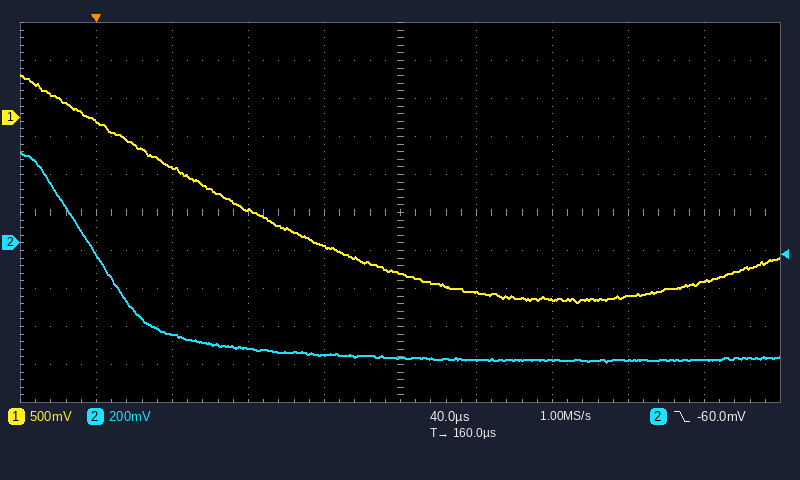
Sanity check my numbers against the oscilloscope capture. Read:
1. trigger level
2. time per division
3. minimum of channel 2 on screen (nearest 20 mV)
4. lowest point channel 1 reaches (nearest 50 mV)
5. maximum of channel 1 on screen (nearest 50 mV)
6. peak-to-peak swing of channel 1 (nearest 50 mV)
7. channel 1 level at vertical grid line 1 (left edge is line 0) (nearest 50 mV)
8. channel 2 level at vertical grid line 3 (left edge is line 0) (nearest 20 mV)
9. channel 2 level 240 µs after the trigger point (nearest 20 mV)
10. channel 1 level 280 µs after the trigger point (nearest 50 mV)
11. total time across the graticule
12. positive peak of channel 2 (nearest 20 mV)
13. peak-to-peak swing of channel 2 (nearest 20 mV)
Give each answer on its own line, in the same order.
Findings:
-60.0 mV
40 µs
-620 mV
-2.45 V
550 mV
3.00 V
-50 mV
-560 mV
-620 mV
-2.35 V
400 µs
480 mV
1.10 V
